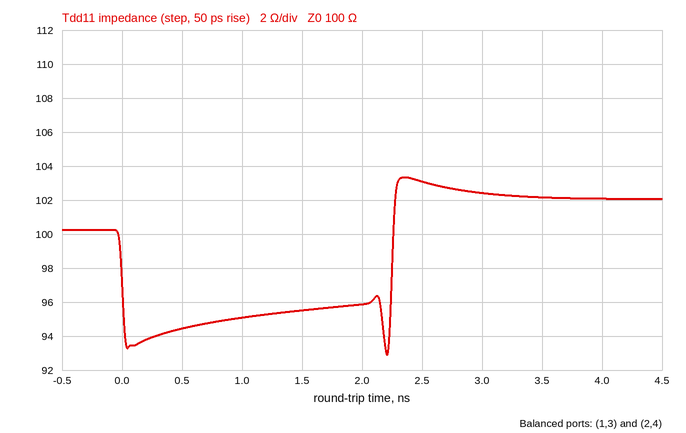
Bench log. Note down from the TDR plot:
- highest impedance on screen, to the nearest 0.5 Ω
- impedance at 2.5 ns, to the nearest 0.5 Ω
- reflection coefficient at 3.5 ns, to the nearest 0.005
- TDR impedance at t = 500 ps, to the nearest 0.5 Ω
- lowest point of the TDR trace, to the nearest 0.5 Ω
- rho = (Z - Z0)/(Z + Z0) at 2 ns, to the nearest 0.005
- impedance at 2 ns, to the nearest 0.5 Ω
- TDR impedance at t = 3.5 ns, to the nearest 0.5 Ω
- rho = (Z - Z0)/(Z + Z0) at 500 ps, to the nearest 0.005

103.5 Ω
103.0 Ω
+0.010
94.5 Ω
93.0 Ω
-0.020
96.0 Ω
102.0 Ω
-0.030
